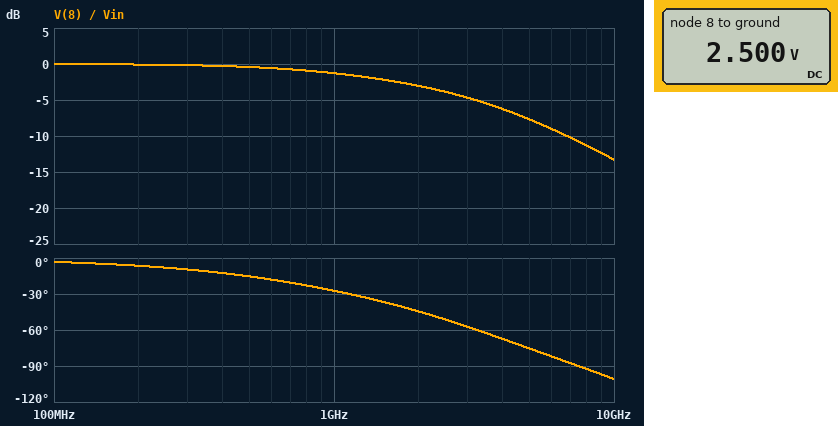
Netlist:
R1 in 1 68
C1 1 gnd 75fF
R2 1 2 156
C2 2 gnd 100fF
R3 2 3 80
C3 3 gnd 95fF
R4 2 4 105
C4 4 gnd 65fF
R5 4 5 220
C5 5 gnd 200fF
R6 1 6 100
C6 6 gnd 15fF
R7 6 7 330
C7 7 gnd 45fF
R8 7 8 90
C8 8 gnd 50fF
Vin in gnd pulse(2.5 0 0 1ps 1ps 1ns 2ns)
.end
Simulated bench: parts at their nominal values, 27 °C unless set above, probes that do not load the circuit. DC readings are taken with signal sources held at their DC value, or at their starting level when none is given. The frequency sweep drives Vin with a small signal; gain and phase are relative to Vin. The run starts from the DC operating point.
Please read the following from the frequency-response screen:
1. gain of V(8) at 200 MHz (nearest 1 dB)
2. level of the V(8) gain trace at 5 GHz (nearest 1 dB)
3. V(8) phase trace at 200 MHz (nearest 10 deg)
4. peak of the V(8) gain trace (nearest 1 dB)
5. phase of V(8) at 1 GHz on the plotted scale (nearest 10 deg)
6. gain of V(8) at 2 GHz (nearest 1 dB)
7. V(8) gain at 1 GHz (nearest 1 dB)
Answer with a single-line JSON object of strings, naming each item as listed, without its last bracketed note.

{"gain of V(8) at 200 MHz": "0 dB", "level of the V(8) gain trace at 5 GHz": "-8 dB", "V(8) phase trace at 200 MHz": "-10 deg", "peak of the V(8) gain trace": "0 dB", "phase of V(8) at 1 GHz on the plotted scale": "-30 deg", "gain of V(8) at 2 GHz": "-3 dB", "V(8) gain at 1 GHz": "-1 dB"}
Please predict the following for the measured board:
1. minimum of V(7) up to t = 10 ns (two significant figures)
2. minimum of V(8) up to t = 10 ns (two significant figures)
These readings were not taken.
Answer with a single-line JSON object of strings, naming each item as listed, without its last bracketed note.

{"minimum of V(7) up to t = 10 ns": "1.1 mV", "minimum of V(8) up to t = 10 ns": "1.1 mV"}
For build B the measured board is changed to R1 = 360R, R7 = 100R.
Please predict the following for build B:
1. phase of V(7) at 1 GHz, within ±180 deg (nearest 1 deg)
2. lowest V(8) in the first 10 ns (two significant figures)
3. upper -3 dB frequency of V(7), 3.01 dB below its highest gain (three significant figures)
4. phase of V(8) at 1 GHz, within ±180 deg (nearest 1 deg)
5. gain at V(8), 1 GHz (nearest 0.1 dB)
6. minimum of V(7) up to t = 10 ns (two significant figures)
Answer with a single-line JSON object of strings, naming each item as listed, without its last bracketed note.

{"phase of V(7) at 1 GHz, within ±180 deg": "-44 deg", "lowest V(8) in the first 10 ns": "81 mV", "upper -3 dB frequency of V(7), 3.01 dB below its highest gain": "561 MHz", "phase of V(8) at 1 GHz, within ±180 deg": "-46 deg", "gain at V(8), 1 GHz": "-5.5 dB", "minimum of V(7) up to t = 10 ns": "80 mV"}
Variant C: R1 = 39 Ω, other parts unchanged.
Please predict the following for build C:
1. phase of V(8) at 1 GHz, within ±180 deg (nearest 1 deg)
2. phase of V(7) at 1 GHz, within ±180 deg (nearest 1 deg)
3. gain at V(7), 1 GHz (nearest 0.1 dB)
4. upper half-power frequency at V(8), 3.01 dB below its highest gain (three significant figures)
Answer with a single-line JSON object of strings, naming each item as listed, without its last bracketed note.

{"phase of V(8) at 1 GHz, within ±180 deg": "-23 deg", "phase of V(7) at 1 GHz, within ±180 deg": "-21 deg", "gain at V(7), 1 GHz": "-0.8 dB", "upper half-power frequency at V(8), 3.01 dB below its highest gain": "2.55 GHz"}
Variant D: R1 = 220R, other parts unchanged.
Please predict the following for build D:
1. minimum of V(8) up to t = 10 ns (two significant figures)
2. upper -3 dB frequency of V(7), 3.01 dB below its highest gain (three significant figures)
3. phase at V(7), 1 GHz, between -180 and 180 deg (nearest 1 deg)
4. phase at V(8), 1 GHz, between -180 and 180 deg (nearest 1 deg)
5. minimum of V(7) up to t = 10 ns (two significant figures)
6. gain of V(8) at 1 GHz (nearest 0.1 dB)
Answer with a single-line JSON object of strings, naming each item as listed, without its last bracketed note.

{"minimum of V(8) up to t = 10 ns": "26 mV", "upper -3 dB frequency of V(7), 3.01 dB below its highest gain": "829 MHz", "phase at V(7), 1 GHz, between -180 and 180 deg": "-42 deg", "phase at V(8), 1 GHz, between -180 and 180 deg": "-44 deg", "minimum of V(7) up to t = 10 ns": "25 mV", "gain of V(8) at 1 GHz": "-3.7 dB"}
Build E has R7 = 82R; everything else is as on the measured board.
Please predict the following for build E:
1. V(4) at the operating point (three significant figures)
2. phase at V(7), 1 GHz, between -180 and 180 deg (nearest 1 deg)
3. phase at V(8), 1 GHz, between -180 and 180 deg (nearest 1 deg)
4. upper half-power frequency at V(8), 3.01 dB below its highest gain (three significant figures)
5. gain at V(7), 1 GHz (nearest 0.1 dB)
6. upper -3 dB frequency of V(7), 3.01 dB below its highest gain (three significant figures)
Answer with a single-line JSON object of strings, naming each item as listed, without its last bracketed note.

{"V(4) at the operating point": "2.50 V", "phase at V(7), 1 GHz, between -180 and 180 deg": "-18 deg", "phase at V(8), 1 GHz, between -180 and 180 deg": "-19 deg", "upper half-power frequency at V(8), 3.01 dB below its highest gain": "3.02 GHz", "gain at V(7), 1 GHz": "-1.0 dB", "upper -3 dB frequency of V(7), 3.01 dB below its highest gain": "3.06 GHz"}
